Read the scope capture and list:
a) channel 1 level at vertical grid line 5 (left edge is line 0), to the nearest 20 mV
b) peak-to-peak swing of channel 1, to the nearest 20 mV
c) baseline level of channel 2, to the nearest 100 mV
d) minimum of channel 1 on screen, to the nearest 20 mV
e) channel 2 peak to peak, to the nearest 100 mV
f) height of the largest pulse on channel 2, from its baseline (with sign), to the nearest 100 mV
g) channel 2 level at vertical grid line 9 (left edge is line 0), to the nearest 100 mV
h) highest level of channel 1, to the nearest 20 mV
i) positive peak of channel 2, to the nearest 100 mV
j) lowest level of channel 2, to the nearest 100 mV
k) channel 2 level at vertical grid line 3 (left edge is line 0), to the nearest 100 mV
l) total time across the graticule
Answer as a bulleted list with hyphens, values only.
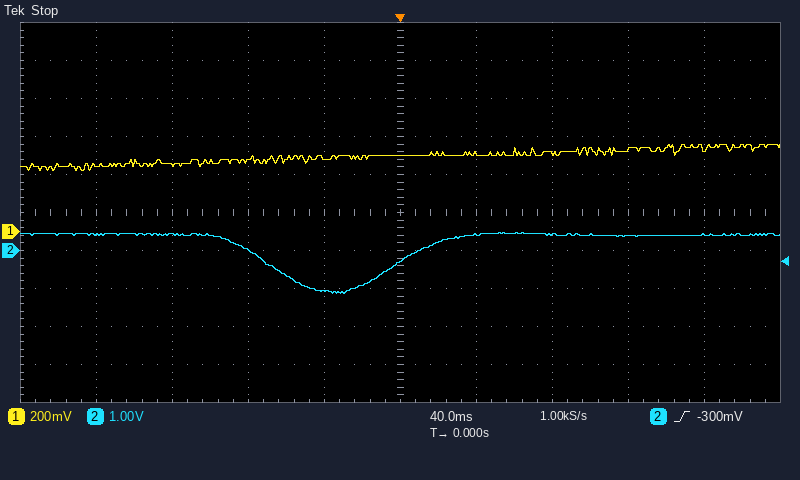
- 400 mV
- 140 mV
- 400 mV
- 320 mV
- 1.6 V
- -1.5 V
- 400 mV
- 460 mV
- 500 mV
- -1.1 V
- 0.0 V
- 400 ms
